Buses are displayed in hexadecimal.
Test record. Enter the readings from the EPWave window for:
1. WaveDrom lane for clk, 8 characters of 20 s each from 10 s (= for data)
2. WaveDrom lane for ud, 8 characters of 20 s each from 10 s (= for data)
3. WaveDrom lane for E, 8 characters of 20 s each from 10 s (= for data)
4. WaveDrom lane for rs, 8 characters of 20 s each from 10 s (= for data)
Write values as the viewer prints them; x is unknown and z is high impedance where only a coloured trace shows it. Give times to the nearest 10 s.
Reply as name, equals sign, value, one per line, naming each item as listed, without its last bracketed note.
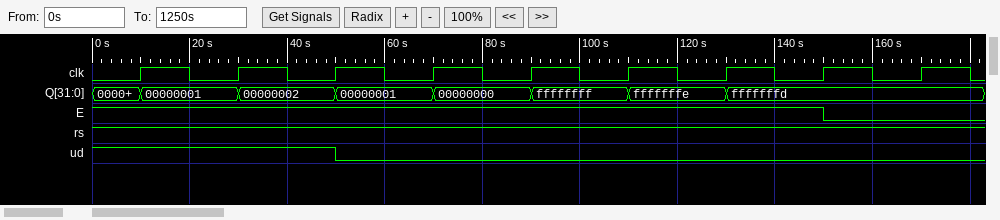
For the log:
WaveDrom lane for clk, 8 characters of 20 s each from 10 s = {name: 'clk', wave: 'p.......'}
WaveDrom lane for ud, 8 characters of 20 s each from 10 s = {name: 'ud', wave: '1.0.....'}
WaveDrom lane for E, 8 characters of 20 s each from 10 s = {name: 'E', wave: '1......0'}
WaveDrom lane for rs, 8 characters of 20 s each from 10 s = {name: 'rs', wave: '1.......'}
